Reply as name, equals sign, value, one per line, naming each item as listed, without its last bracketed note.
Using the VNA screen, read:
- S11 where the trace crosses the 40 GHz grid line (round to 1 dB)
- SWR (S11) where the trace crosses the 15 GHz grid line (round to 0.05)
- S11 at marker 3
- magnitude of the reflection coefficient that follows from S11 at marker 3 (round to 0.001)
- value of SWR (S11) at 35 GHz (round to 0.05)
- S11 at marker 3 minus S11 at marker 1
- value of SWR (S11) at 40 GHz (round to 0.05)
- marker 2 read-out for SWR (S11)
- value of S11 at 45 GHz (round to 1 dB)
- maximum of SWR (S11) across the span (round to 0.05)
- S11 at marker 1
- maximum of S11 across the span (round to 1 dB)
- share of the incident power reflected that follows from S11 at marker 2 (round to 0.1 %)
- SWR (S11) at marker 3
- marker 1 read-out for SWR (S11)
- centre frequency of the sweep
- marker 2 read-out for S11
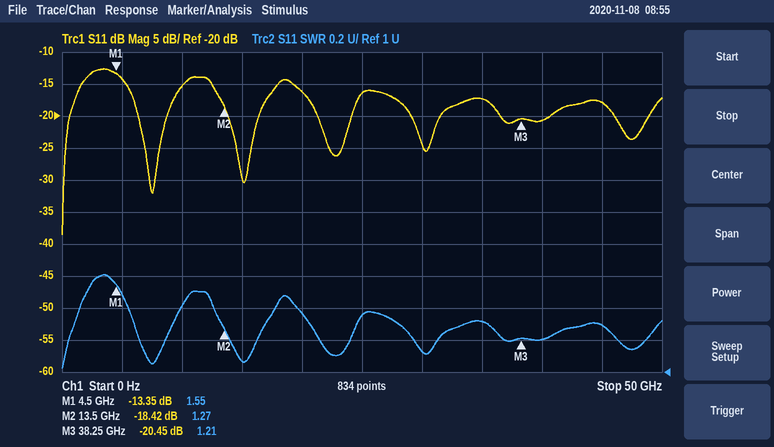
S11 where the trace crosses the 40 GHz grid line = -21 dB
SWR (S11) where the trace crosses the 15 GHz grid line = 1.05
S11 at marker 3 = -20.45 dB
magnitude of the reflection coefficient that follows from S11 at marker 3 = 0.095
value of SWR (S11) at 35 GHz = 1.30
S11 at marker 3 minus S11 at marker 1 = -7.10 dB
value of SWR (S11) at 40 GHz = 1.20
marker 2 read-out for SWR = 1.27
value of S11 at 45 GHz = -18 dB
maximum of SWR (S11) across the span = 1.60
S11 at marker 1 = -13.35 dB
maximum of S11 across the span = -13 dB
share of the incident power reflected that follows from S11 at marker 2 = 1.4 %
SWR (S11) at marker 3 = 1.21
marker 1 read-out for SWR = 1.55
centre frequency of the sweep = 25 GHz
marker 2 read-out for S11 = -18.42 dB
